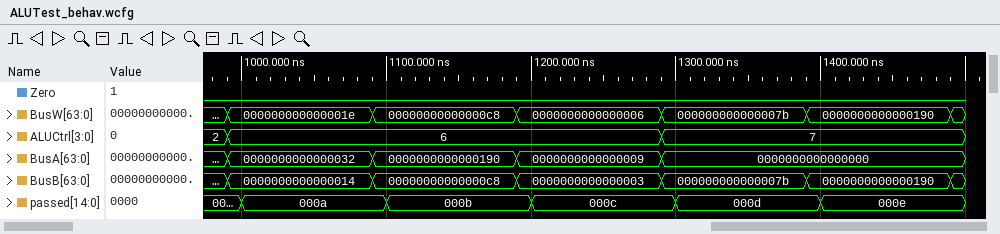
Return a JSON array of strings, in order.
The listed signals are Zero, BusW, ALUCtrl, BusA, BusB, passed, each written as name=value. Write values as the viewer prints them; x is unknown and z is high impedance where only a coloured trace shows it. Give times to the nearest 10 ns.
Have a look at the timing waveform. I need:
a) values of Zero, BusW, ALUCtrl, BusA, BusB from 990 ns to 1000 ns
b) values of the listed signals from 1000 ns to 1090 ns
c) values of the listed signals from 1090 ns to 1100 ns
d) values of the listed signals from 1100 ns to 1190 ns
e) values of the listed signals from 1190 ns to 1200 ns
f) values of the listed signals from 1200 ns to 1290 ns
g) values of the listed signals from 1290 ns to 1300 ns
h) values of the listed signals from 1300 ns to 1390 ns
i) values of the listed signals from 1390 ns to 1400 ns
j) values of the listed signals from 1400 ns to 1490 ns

["Zero=0, BusW=000000000000001e, ALUCtrl=6, BusA=0000000000000032, BusB=0000000000000014", "Zero=0, BusW=000000000000001e, ALUCtrl=6, BusA=0000000000000032, BusB=0000000000000014, passed=000a", "Zero=0, BusW=00000000000000c8, ALUCtrl=6, BusA=0000000000000190, BusB=00000000000000c8, passed=000a", "Zero=0, BusW=00000000000000c8, ALUCtrl=6, BusA=0000000000000190, BusB=00000000000000c8, passed=000b", "Zero=0, BusW=0000000000000006, ALUCtrl=6, BusA=0000000000000009, BusB=0000000000000003, passed=000b", "Zero=0, BusW=0000000000000006, ALUCtrl=6, BusA=0000000000000009, BusB=0000000000000003, passed=000c", "Zero=0, BusW=000000000000007b, ALUCtrl=7, BusA=0000000000000000, BusB=000000000000007b, passed=000c", "Zero=0, BusW=000000000000007b, ALUCtrl=7, BusA=0000000000000000, BusB=000000000000007b, passed=000d", "Zero=0, BusW=0000000000000190, ALUCtrl=7, BusA=0000000000000000, BusB=0000000000000190, passed=000d", "Zero=0, BusW=0000000000000190, ALUCtrl=7, BusA=0000000000000000, BusB=0000000000000190, passed=000e"]
